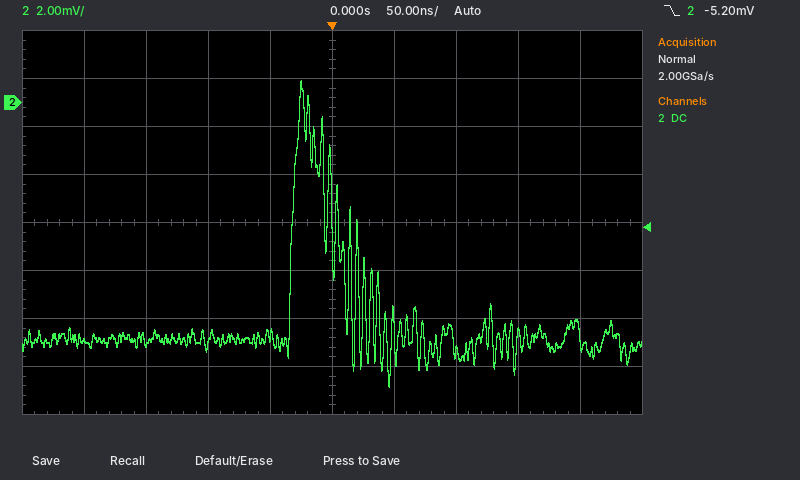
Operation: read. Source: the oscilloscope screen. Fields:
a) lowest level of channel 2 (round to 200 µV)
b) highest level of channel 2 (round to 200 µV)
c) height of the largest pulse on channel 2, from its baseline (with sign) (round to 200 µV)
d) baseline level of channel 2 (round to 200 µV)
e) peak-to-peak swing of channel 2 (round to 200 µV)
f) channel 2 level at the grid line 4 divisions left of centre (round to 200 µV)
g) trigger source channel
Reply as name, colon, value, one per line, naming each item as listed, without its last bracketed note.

lowest level of channel 2: -11.8 mV
highest level of channel 2: 1.0 mV
height of the largest pulse on channel 2, from its baseline (with sign): +10.8 mV
baseline level of channel 2: -9.8 mV
peak-to-peak swing of channel 2: 12.8 mV
channel 2 level at the grid line 4 divisions left of centre: -10.0 mV
trigger source channel: channel 2
